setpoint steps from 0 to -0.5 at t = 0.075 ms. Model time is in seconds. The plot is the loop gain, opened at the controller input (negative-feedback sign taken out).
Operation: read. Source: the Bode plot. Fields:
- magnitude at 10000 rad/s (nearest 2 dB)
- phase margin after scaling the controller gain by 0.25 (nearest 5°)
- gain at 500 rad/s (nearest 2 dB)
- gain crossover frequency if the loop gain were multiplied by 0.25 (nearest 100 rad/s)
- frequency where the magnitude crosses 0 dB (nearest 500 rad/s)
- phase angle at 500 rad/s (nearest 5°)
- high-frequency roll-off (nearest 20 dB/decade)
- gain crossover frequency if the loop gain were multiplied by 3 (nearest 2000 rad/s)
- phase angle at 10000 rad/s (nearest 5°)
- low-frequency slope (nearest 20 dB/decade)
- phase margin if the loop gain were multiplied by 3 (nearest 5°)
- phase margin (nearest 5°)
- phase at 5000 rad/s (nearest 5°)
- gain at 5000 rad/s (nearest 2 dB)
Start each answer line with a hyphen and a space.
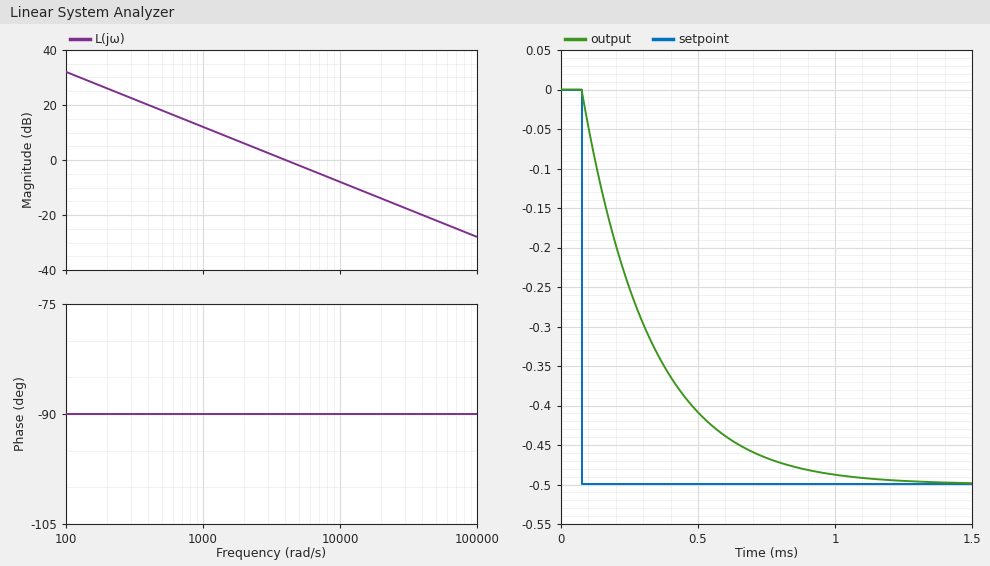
- -8 dB
- 90°
- 18 dB
- 1000 rad/s
- 4000 rad/s
- -90°
- -20 dB/decade
- 12000 rad/s
- -90°
- -20 dB/decade
- 90°
- 90°
- -90°
- -2 dB
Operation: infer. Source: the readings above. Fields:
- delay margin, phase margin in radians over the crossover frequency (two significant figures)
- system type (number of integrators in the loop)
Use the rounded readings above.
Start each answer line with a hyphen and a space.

- 0.00039 s
- 1
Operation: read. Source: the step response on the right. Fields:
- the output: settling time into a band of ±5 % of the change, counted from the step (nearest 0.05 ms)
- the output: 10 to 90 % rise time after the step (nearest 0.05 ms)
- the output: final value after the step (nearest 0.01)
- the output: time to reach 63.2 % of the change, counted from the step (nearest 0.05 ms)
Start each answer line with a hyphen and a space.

- 0.75 ms
- 0.55 ms
- -0.50
- 0.25 ms
